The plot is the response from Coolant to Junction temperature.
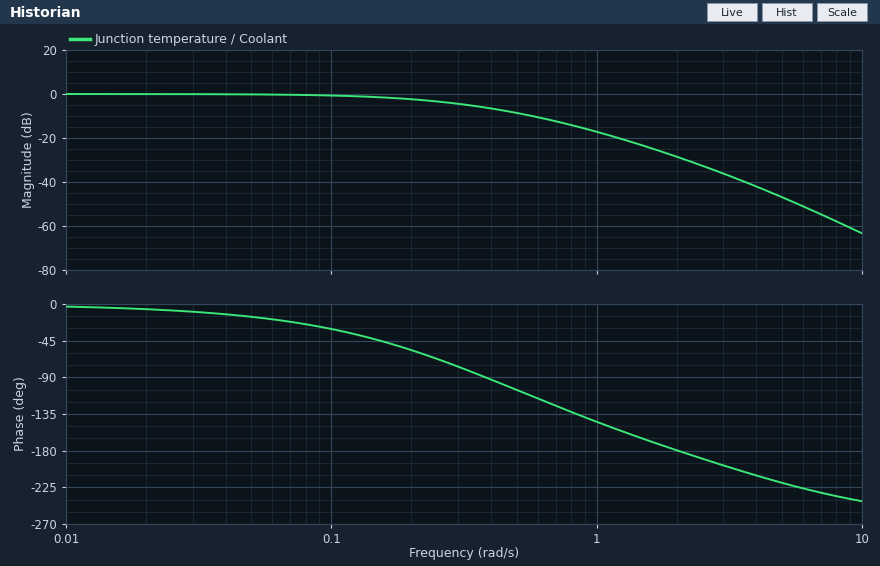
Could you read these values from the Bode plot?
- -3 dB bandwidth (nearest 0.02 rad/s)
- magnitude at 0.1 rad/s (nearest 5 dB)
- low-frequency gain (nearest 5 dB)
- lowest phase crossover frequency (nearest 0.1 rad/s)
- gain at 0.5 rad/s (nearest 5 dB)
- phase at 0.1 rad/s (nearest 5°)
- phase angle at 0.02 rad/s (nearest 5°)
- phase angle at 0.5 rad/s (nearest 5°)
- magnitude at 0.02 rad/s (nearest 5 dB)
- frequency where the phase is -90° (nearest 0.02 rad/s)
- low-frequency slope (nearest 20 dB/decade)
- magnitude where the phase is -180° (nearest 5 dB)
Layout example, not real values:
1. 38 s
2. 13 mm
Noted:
1. 0.24 rad/s
2. 0 dB
3. 0 dB
4. 2.0 rad/s
5. -10 dB
6. -30°
7. -5°
8. -105°
9. 0 dB
10. 0.38 rad/s
11. 0 dB/decade
12. -30 dB
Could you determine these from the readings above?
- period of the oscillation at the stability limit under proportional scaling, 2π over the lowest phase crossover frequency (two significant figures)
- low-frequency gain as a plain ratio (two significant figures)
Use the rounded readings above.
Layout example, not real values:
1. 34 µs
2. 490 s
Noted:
1. 3.1 s
2. 1.0
